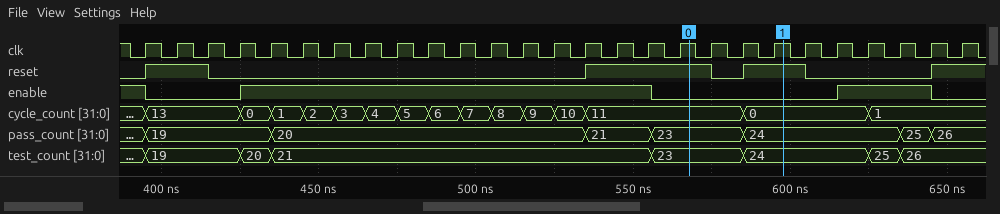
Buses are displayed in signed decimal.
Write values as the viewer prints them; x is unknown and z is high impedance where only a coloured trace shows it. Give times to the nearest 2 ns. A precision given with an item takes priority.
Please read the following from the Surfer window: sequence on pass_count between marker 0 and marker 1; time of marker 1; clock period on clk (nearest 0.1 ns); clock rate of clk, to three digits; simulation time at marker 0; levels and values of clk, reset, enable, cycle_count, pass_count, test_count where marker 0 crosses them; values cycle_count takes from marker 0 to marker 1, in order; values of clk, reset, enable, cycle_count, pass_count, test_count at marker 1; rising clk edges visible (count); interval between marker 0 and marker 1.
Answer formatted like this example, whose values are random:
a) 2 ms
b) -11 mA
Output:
a) 23, 24
b) 598 ns
c) 10 ns
d) 100 MHz
e) 568 ns
f) clk=1, reset=1, enable=0, cycle_count=11, pass_count=23, test_count=23
g) 11, 0
h) clk=1, reset=1, enable=0, cycle_count=0, pass_count=24, test_count=24
i) 27
j) 30 ns
